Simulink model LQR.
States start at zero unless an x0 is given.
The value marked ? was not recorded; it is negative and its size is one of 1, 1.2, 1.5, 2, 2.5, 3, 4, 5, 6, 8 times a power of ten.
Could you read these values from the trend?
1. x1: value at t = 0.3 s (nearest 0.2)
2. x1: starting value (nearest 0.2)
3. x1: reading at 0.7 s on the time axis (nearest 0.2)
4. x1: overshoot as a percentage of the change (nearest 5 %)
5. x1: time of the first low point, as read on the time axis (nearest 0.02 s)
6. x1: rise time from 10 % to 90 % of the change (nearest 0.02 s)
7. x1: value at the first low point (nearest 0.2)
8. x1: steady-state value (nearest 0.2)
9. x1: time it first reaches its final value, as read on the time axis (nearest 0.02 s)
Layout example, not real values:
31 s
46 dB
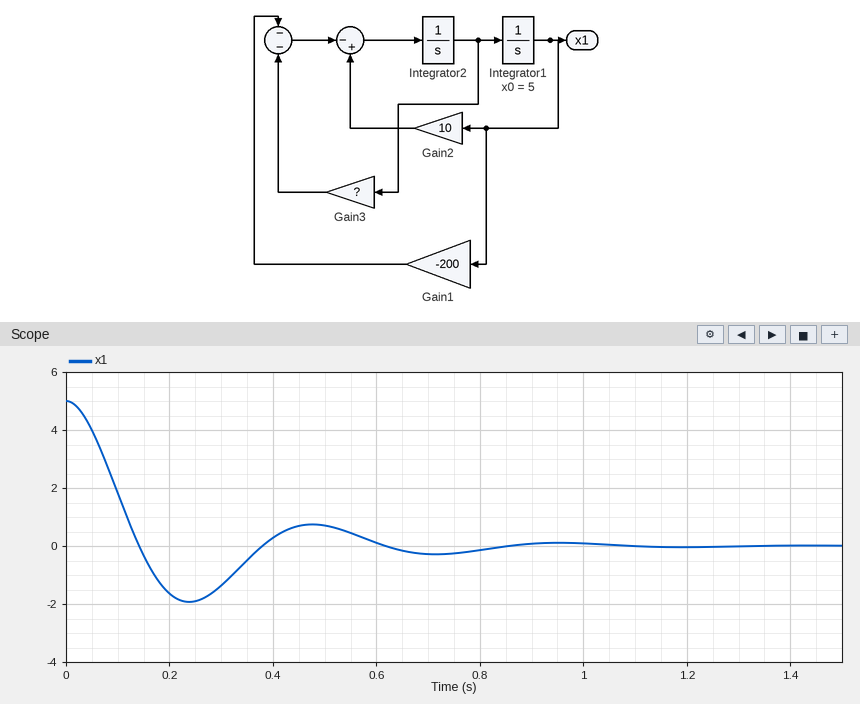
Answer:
-1.4
5.0
-0.2
40 %
0.24 s
0.10 s
-2.0
0.0
0.14 s
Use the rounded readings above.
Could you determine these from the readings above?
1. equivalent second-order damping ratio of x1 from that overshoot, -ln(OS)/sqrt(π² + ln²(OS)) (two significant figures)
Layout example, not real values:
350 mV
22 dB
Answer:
0.28
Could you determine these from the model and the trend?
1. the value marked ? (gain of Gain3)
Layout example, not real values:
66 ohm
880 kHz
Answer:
-8
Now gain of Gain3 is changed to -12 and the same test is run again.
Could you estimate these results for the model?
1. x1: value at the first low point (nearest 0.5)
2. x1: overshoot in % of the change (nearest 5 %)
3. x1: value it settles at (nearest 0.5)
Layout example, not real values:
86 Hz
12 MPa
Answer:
-1.0
20 %
0.0
